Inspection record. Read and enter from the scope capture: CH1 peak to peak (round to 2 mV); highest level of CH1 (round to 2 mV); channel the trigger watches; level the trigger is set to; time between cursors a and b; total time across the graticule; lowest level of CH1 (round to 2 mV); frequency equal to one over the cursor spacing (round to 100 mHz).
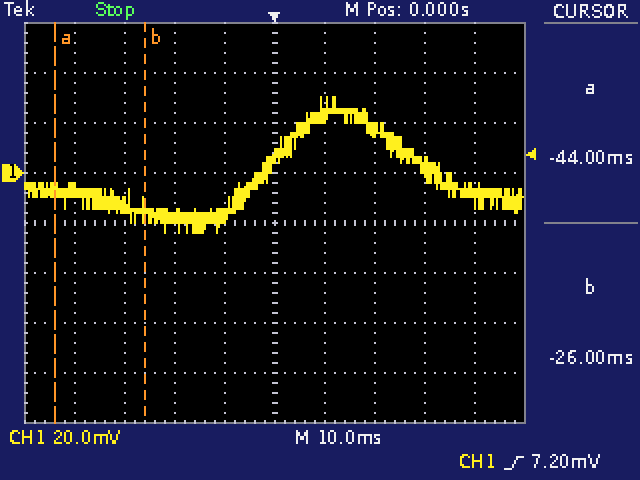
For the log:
54 mV
30 mV
CH1
7.20 mV
18 ms
100 ms
-24 mV
55.6 Hz
